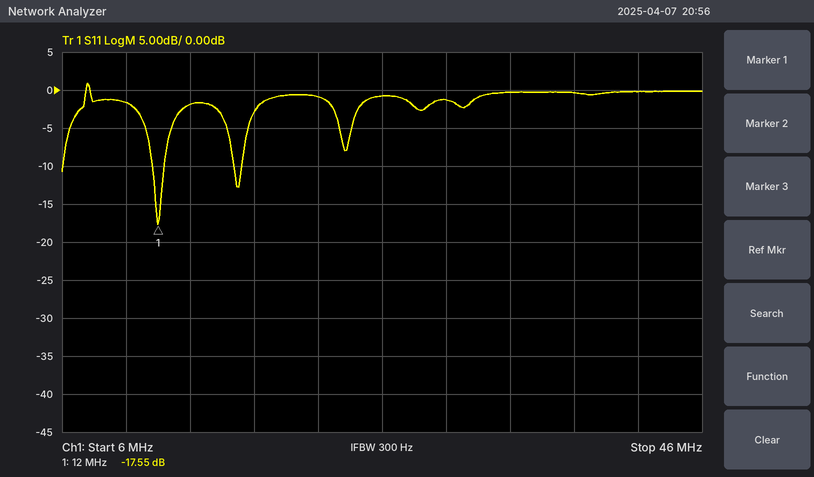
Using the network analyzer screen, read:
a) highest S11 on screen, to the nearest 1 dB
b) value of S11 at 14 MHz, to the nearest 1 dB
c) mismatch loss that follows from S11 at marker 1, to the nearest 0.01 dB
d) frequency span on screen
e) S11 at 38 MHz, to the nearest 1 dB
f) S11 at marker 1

1 dB
-2 dB
0.08 dB
40 MHz
0 dB
-17.55 dB
